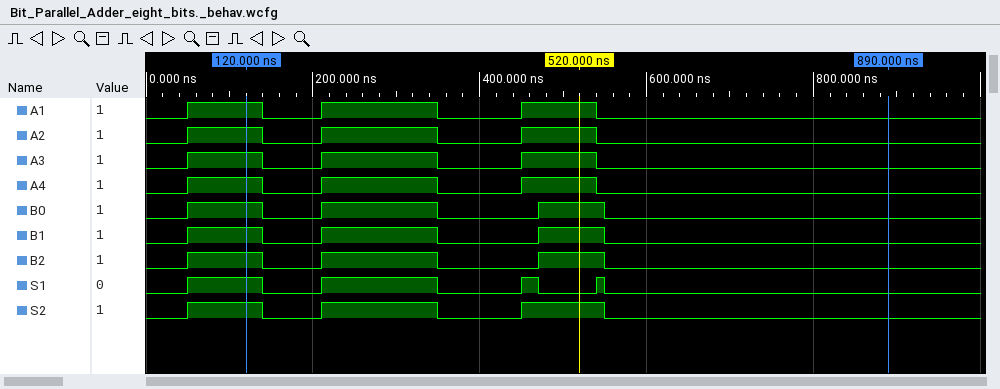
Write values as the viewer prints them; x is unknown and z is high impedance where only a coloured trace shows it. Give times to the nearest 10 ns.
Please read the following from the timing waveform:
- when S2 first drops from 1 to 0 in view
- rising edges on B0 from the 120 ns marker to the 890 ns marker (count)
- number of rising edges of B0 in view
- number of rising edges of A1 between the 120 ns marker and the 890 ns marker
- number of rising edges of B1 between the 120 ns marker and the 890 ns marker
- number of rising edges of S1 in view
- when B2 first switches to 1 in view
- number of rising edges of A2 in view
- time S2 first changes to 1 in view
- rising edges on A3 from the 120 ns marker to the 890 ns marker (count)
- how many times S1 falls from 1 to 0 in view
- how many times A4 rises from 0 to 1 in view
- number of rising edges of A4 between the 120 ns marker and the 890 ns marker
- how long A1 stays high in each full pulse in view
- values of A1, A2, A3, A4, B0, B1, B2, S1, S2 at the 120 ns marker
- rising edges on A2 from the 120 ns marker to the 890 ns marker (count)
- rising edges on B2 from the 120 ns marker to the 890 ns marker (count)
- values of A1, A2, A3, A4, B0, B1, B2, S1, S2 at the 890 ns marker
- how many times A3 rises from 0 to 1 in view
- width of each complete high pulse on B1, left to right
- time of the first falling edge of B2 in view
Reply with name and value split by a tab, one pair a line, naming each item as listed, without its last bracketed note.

when S2 first drops from 1 to 0 in view	140 ns
rising edges on B0 from the 120 ns marker to the 890 ns marker	2
number of rising edges of B0 in view	3
number of rising edges of A1 between the 120 ns marker and the 890 ns marker	2
number of rising edges of B1 between the 120 ns marker and the 890 ns marker	2
number of rising edges of S1 in view	4
when B2 first switches to 1 in view	50 ns
number of rising edges of A2 in view	3
time S2 first changes to 1 in view	50 ns
rising edges on A3 from the 120 ns marker to the 890 ns marker	2
how many times S1 falls from 1 to 0 in view	4
how many times A4 rises from 0 to 1 in view	3
number of rising edges of A4 between the 120 ns marker and the 890 ns marker	2
how long A1 stays high in each full pulse in view	90 ns, 140 ns, 90 ns
values of A1, A2, A3, A4, B0, B1, B2, S1, S2 at the 120 ns marker	A1=1, A2=1, A3=1, A4=1, B0=1, B1=1, B2=1, S1=1, S2=1
rising edges on A2 from the 120 ns marker to the 890 ns marker	2
rising edges on B2 from the 120 ns marker to the 890 ns marker	2
values of A1, A2, A3, A4, B0, B1, B2, S1, S2 at the 890 ns marker	A1=0, A2=0, A3=0, A4=0, B0=0, B1=0, B2=0, S1=0, S2=0
how many times A3 rises from 0 to 1 in view	3
width of each complete high pulse on B1, left to right	90 ns, 140 ns, 80 ns
time of the first falling edge of B2 in view	140 ns
